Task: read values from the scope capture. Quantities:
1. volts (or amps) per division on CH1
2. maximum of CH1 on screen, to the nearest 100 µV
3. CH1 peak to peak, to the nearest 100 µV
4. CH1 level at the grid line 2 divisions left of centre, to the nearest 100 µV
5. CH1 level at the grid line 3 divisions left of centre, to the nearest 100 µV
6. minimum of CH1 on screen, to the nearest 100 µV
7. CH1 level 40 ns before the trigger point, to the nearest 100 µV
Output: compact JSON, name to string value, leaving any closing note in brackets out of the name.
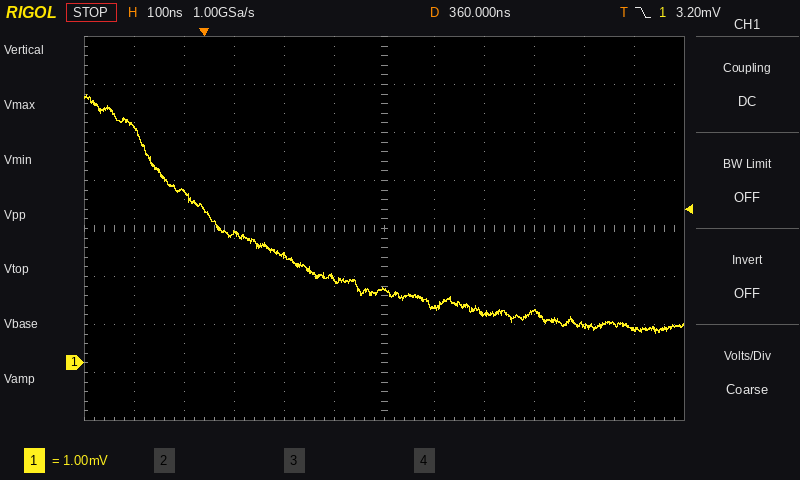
{"volts (or amps) per division on CH1": "1 mV", "maximum of CH1 on screen, to the nearest 100 µV": "5.6 mV", "CH1 peak to peak, to the nearest 100 µV": "5.0 mV", "CH1 level at the grid line 2 divisions left of centre, to the nearest 100 µV": "2.2 mV", "CH1 level at the grid line 3 divisions left of centre, to the nearest 100 µV": "2.7 mV", "minimum of CH1 on screen, to the nearest 100 µV": "600 µV", "CH1 level 40 ns before the trigger point, to the nearest 100 µV": "3.6 mV"}
